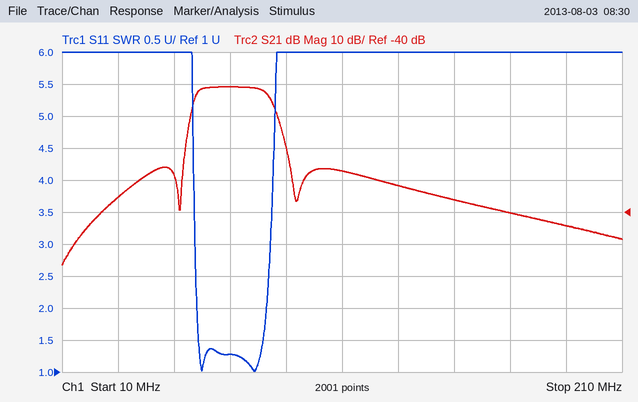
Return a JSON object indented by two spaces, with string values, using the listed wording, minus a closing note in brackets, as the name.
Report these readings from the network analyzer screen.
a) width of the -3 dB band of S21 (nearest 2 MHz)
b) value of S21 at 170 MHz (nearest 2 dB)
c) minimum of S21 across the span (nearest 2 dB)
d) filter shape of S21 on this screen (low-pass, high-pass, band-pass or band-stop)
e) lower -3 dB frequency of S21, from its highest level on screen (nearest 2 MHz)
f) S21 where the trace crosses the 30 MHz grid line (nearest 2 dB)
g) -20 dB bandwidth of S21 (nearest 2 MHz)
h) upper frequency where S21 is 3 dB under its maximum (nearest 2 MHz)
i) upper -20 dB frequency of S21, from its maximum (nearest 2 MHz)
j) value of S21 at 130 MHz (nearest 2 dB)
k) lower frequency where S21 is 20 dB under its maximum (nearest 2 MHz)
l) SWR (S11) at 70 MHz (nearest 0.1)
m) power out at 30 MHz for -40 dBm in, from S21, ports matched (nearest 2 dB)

{
  "width of the -3 dB band of S21": "26 MHz",
  "value of S21 at 170 MHz": "-40 dB",
  "minimum of S21 across the span": "-56 dB",
  "filter shape of S21 on this screen": "band-pass",
  "lower -3 dB frequency of S21, from its highest level on screen": "58 MHz",
  "S21 where the trace crosses the 30 MHz grid line": "-36 dB",
  "-20 dB bandwidth of S21": "36 MHz",
  "upper frequency where S21 is 3 dB under its maximum": "84 MHz",
  "upper -20 dB frequency of S21, from its maximum": "90 MHz",
  "value of S21 at 130 MHz": "-32 dB",
  "lower frequency where S21 is 20 dB under its maximum": "54 MHz",
  "SWR (S11) at 70 MHz": "1.3",
  "power out at 30 MHz for -40 dBm in, from S21, ports matched": "-76 dBm"
}
